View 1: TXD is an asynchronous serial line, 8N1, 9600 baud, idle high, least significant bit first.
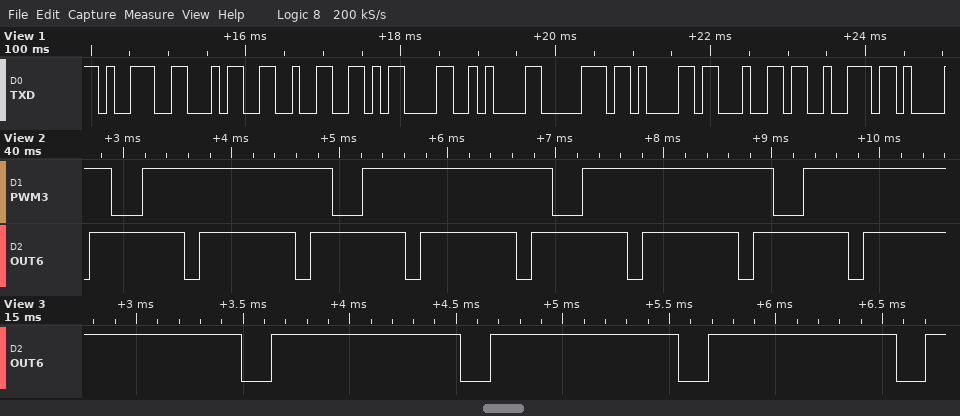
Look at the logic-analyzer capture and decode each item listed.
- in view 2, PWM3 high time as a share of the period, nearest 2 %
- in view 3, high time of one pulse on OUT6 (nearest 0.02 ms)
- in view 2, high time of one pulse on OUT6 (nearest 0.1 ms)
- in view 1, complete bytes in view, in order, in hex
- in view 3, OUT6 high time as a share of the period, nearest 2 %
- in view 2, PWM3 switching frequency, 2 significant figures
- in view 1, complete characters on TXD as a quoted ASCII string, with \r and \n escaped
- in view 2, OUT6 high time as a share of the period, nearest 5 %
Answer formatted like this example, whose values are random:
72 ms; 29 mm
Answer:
86 %; 0.88 ms; 0.9 ms; 39 34 32 0D 0A 70 61 64 72; 86 %; 490 Hz; "942\r\npadr"; 85 %
